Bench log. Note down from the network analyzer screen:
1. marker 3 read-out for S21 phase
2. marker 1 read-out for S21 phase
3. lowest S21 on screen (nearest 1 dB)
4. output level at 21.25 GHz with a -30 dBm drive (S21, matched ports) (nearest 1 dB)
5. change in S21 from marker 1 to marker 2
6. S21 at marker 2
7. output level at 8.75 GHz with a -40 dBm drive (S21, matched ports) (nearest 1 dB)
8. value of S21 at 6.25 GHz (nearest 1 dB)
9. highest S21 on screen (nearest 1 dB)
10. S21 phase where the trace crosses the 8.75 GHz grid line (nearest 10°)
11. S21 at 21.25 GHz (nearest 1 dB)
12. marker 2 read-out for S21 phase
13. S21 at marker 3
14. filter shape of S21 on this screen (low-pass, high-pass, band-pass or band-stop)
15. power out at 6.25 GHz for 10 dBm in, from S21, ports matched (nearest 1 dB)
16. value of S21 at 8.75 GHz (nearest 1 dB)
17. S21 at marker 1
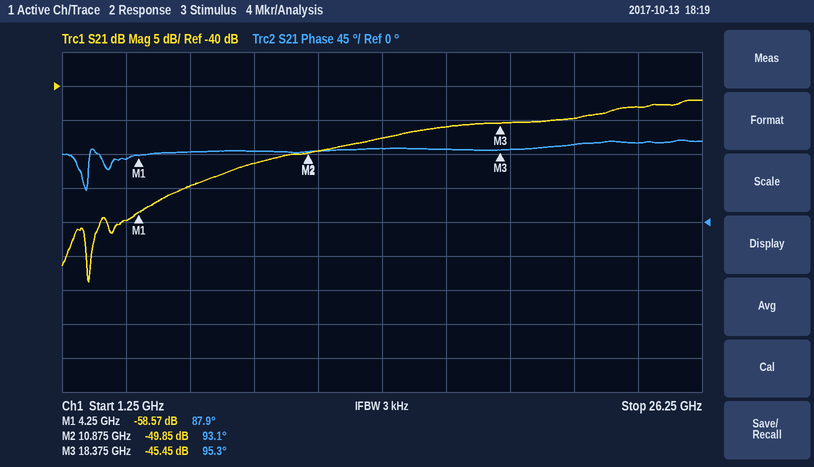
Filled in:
95.3°
87.9°
-69 dB
-75 dBm
8.72 dB
-49.85 dB
-91 dBm
-55 dB
-42 dB
90°
-45 dB
93.1°
-45.45 dB
high-pass
-45 dBm
-51 dB
-58.57 dB
